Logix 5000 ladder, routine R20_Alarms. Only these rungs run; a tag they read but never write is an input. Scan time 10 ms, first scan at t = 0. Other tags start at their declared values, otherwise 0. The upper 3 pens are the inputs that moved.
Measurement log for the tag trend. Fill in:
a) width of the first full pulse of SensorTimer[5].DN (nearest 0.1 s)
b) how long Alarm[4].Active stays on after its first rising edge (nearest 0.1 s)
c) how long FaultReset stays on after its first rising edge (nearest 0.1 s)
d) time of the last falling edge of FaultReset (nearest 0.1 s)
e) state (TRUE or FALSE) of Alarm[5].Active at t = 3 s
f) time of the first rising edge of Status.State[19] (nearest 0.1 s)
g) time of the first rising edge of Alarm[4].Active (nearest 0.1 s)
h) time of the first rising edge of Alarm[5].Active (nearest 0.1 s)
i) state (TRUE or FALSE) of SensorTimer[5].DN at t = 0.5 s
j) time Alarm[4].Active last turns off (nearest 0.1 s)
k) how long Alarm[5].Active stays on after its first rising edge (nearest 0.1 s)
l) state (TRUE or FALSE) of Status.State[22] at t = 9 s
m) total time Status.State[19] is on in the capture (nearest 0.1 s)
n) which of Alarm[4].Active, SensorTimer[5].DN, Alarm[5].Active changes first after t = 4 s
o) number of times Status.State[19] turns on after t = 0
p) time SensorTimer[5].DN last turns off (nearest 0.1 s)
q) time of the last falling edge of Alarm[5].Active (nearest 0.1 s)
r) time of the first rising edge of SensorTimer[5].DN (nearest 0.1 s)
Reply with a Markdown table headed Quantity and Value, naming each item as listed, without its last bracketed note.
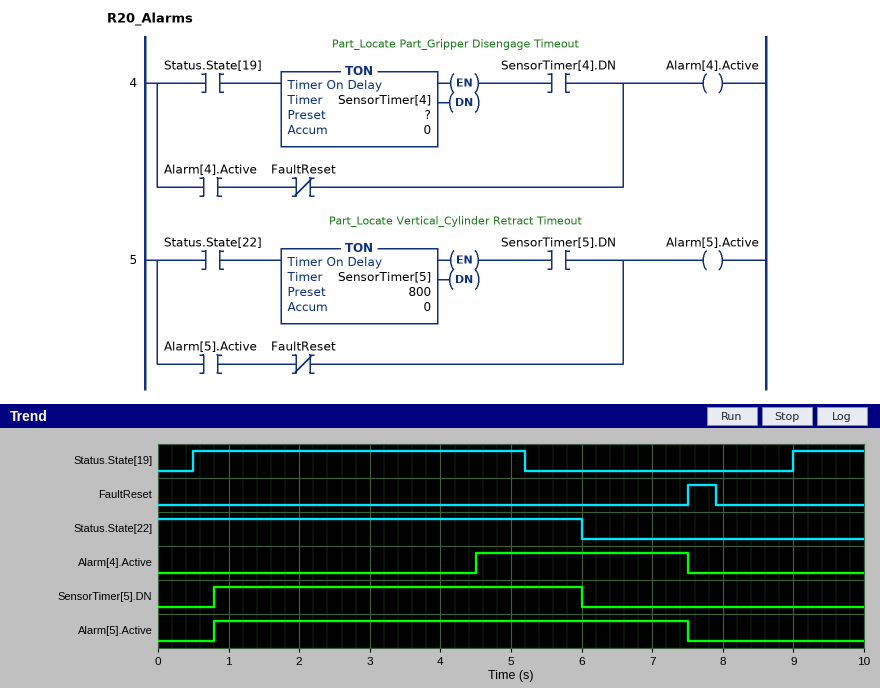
| Quantity | Value |
|---|---|
| width of the first full pulse of SensorTimer[5].DN | 5.2 s |
| how long Alarm[4].Active stays on after its first rising edge | 3.0 s |
| how long FaultReset stays on after its first rising edge | 0.4 s |
| time of the last falling edge of FaultReset | 7.9 s |
| state (TRUE or FALSE) of Alarm[5].Active at t = 3 s | TRUE |
| time of the first rising edge of Status.State[19] | 0.5 s |
| time of the first rising edge of Alarm[4].Active | 4.5 s |
| time of the first rising edge of Alarm[5].Active | 0.8 s |
| state (TRUE or FALSE) of SensorTimer[5].DN at t = 0.5 s | FALSE |
| time Alarm[4].Active last turns off | 7.5 s |
| how long Alarm[5].Active stays on after its first rising edge | 6.7 s |
| state (TRUE or FALSE) of Status.State[22] at t = 9 s | FALSE |
| total time Status.State[19] is on in the capture | 5.7 s |
| which of Alarm[4].Active, SensorTimer[5].DN, Alarm[5].Active changes first after t = 4 s | Alarm[4].Active |
| number of times Status.State[19] turns on after t = 0 | 2 |
| time SensorTimer[5].DN last turns off | 6.0 s |
| time of the last falling edge of Alarm[5].Active | 7.5 s |
| time of the first rising edge of SensorTimer[5].DN | 0.8 s |
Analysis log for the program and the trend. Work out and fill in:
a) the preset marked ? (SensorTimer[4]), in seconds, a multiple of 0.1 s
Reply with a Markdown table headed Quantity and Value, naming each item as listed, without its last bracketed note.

| Quantity | Value |
|---|---|
| the preset marked ? (SensorTimer[4]), in seconds, a multiple of 0.1 s | 4.0 s |
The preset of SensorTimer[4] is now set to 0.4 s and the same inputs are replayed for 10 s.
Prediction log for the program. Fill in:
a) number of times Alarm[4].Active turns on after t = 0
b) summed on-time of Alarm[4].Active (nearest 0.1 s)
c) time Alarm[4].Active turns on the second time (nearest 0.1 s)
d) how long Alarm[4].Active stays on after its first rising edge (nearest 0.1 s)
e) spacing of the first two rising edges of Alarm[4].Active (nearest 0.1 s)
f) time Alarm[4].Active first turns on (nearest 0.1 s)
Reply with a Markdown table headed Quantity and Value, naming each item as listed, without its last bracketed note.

| Quantity | Value |
|---|---|
| number of times Alarm[4].Active turns on after t = 0 | 2 |
| summed on-time of Alarm[4].Active | 7.2 s |
| time Alarm[4].Active turns on the second time | 9.4 s |
| how long Alarm[4].Active stays on after its first rising edge | 6.6 s |
| spacing of the first two rising edges of Alarm[4].Active | 8.5 s |
| time Alarm[4].Active first turns on | 0.9 s |
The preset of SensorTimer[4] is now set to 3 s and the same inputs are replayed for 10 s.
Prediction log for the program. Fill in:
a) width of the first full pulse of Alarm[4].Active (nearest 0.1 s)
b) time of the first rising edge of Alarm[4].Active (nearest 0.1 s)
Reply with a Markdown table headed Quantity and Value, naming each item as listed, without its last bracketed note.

| Quantity | Value |
|---|---|
| width of the first full pulse of Alarm[4].Active | 4.0 s |
| time of the first rising edge of Alarm[4].Active | 3.5 s |
